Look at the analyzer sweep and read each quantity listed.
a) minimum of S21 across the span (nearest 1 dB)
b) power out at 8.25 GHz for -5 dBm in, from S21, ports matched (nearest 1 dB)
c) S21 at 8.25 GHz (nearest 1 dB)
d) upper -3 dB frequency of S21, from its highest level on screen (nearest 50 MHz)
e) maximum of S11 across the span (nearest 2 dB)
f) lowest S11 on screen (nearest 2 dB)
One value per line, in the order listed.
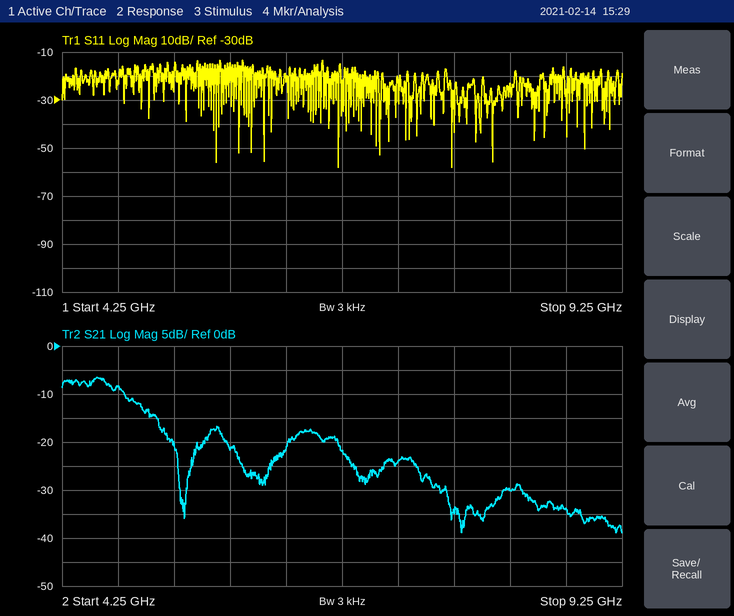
-39 dB
-35 dBm
-30 dB
4.80 GHz
-14 dB
-58 dB
